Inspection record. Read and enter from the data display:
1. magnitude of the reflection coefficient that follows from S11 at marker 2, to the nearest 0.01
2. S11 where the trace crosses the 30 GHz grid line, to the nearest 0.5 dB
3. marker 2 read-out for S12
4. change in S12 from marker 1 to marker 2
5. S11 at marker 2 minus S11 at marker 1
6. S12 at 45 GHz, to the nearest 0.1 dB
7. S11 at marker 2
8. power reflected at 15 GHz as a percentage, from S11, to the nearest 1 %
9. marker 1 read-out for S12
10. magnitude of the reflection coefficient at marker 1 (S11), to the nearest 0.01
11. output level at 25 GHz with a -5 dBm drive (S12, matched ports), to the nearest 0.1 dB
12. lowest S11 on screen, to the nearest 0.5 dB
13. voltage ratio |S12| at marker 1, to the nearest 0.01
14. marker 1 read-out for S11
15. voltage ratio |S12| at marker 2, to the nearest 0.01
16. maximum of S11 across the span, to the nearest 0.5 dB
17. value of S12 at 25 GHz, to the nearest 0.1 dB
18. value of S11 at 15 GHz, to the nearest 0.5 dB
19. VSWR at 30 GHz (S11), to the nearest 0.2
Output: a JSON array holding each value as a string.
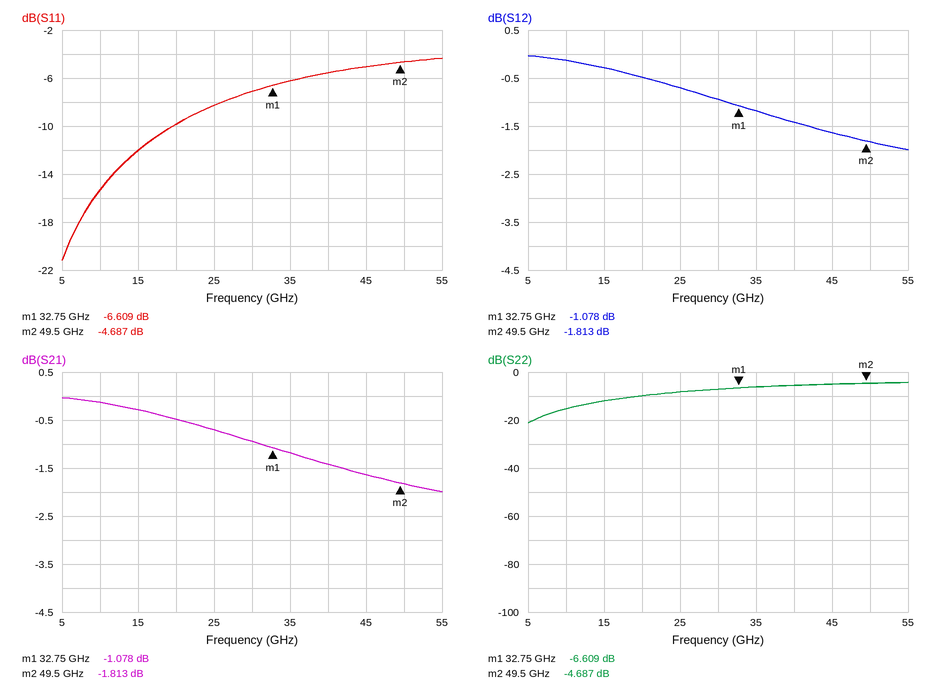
["0.58", "-7.0 dB", "-1.813 dB", "-0.735 dB", "1.922 dB", "-1.6 dB", "-4.687 dB", "6 %", "-1.078 dB", "0.47", "-5.7 dBm", "-21.0 dB", "0.88", "-6.609 dB", "0.81", "-4.5 dB", "-0.7 dB", "-12.0 dB", "2.6"]
